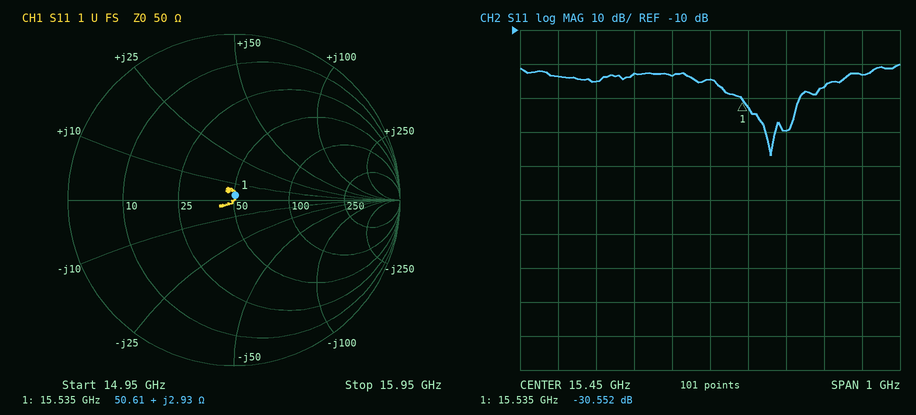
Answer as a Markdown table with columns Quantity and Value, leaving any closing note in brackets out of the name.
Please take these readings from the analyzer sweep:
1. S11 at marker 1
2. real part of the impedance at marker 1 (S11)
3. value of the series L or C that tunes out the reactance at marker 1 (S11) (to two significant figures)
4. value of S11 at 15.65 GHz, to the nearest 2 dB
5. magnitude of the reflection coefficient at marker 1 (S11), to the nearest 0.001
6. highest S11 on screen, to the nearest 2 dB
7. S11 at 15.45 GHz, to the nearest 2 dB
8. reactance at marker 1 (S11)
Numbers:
| Quantity | Value |
|---|---|
| S11 at marker 1 | -30.552 dB |
| real part of the impedance at marker 1 | 50.61 Ω |
| value of the series L or C that tunes out the reactance at marker 1 (S11) | 3.5 pF |
| value of S11 at 15.65 GHz, to the nearest 2 dB | -40 dB |
| magnitude of the reflection coefficient at marker 1 (S11), to the nearest 0.001 | 0.030 |
| highest S11 on screen, to the nearest 2 dB | -20 dB |
| S11 at 15.45 GHz, to the nearest 2 dB | -24 dB |
| reactance at marker 1 | +2.93 Ω |
